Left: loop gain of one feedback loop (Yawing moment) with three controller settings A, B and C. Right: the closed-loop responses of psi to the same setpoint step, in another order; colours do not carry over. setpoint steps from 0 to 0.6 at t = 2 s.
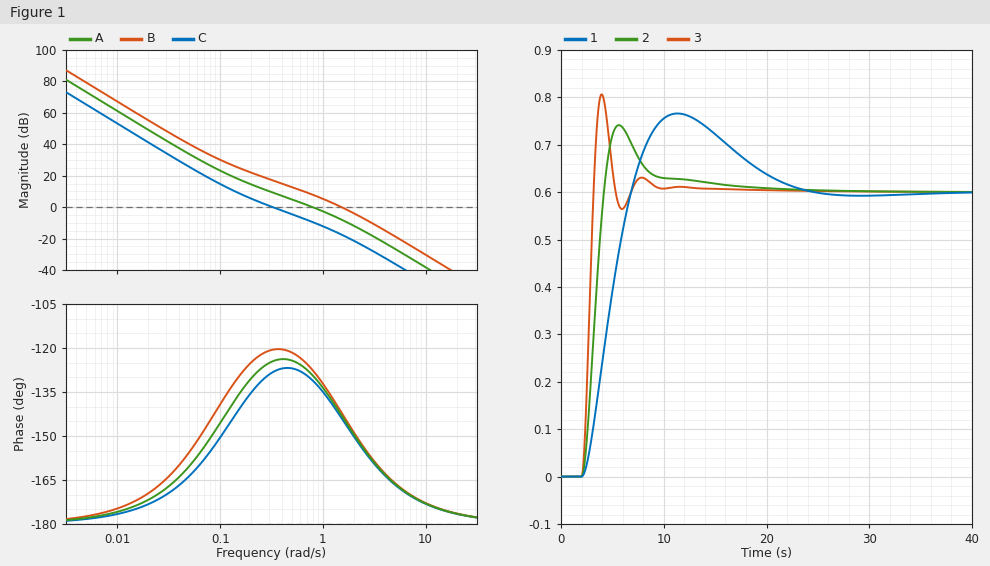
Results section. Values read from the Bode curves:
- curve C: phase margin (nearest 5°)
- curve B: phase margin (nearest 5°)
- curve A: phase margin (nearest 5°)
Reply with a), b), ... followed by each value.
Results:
a) 50°
b) 40°
c) 50°
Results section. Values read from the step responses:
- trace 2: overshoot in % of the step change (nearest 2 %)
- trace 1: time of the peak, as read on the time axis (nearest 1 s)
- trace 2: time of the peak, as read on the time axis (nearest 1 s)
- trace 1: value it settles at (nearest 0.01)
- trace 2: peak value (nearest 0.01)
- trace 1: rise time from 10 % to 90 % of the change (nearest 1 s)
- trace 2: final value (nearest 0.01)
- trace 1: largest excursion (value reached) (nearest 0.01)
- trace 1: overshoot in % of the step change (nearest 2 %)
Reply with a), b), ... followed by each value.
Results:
a) 24 %
b) 11 s
c) 6 s
d) 0.60
e) 0.74
f) 3 s
g) 0.60
h) 0.77
i) 28 %
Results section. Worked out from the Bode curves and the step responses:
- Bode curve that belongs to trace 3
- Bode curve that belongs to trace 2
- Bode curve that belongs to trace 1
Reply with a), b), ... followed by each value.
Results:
a) B
b) A
c) C
